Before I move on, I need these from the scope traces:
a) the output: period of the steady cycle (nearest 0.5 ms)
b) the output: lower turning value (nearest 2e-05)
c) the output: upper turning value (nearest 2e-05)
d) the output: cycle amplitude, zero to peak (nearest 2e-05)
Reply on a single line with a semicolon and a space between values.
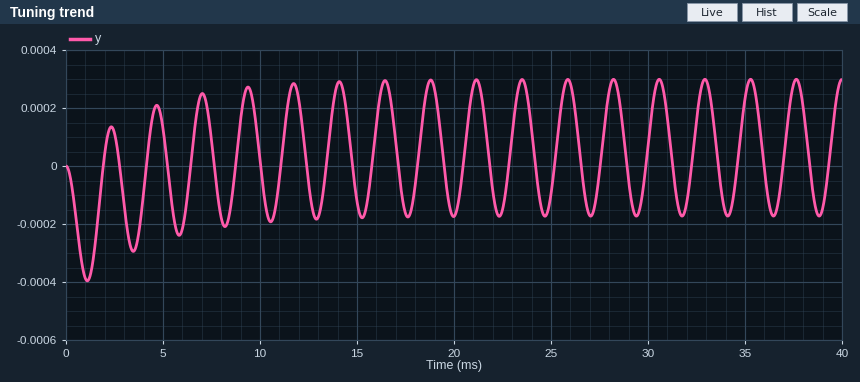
2.5 ms; -0.00018; 0.00030; 0.00024
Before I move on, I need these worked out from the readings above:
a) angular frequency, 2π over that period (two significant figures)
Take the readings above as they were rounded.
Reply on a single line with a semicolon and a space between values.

2.5 rad/ms
